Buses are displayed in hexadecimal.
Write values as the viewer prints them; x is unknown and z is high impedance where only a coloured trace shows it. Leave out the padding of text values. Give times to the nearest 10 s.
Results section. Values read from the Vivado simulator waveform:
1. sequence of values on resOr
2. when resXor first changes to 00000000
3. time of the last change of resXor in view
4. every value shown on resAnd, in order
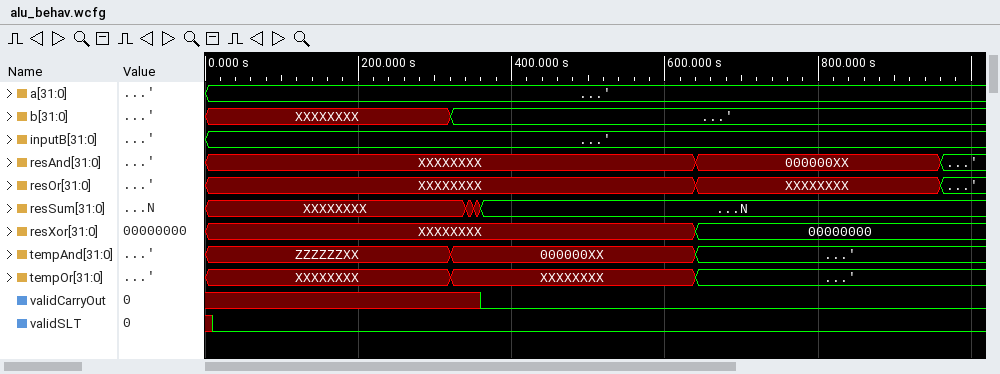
XXXXXXXX, XXXXXXXX, '
640 s
640 s
XXXXXXXX, 000000XX, '
